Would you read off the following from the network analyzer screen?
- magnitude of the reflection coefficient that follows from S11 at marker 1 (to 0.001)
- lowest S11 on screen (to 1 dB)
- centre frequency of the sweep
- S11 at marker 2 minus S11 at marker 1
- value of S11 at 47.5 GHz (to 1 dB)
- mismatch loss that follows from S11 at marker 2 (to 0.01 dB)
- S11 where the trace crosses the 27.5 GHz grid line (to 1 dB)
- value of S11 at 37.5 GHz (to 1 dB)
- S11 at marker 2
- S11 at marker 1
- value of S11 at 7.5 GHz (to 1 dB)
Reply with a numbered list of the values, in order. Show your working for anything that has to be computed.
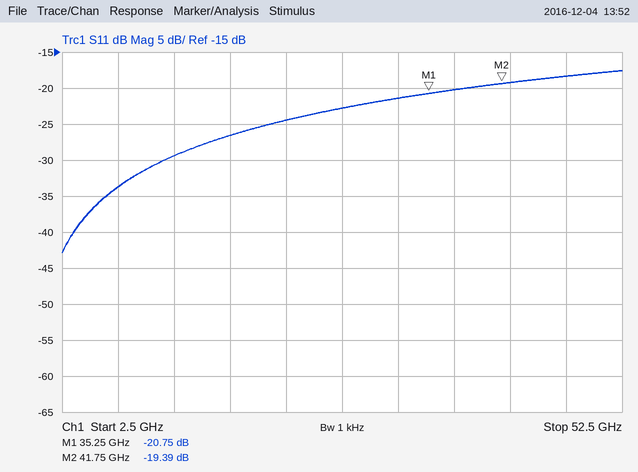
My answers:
1. 10^(-20.75/20) ≈ 0.092
2. -43 dB
3. 27.5 GHz
4. -19.39 − (-20.75) = 1.36 dB
5. -18 dB
6. −10 log10(1 − 10^(-19.39/10)) ≈ 0.05 dB
7. -23 dB
8. -20 dB
9. -19.39 dB
10. -20.75 dB
11. -34 dB
